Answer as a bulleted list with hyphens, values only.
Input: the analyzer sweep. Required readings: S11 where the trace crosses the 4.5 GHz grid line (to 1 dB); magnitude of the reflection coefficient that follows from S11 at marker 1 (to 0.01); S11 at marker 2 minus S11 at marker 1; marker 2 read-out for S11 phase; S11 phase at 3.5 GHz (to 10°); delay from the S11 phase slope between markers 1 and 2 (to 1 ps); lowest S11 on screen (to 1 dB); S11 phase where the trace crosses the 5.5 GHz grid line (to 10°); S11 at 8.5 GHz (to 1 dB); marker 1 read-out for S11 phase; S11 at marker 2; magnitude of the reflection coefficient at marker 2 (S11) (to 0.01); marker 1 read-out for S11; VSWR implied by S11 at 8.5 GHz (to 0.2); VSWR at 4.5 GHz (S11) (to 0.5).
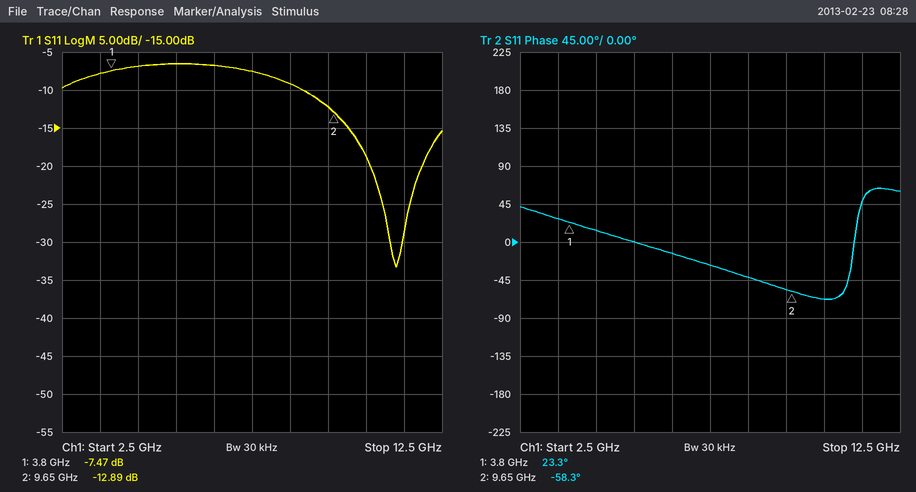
- -7 dB
- 0.42
- -5.42 dB
- -58.3°
- 30°
- 39 ps
- -33 dB
- 0°
- -9 dB
- 23.3°
- -12.89 dB
- 0.23
- -7.47 dB
- 2.0
- 2.5
